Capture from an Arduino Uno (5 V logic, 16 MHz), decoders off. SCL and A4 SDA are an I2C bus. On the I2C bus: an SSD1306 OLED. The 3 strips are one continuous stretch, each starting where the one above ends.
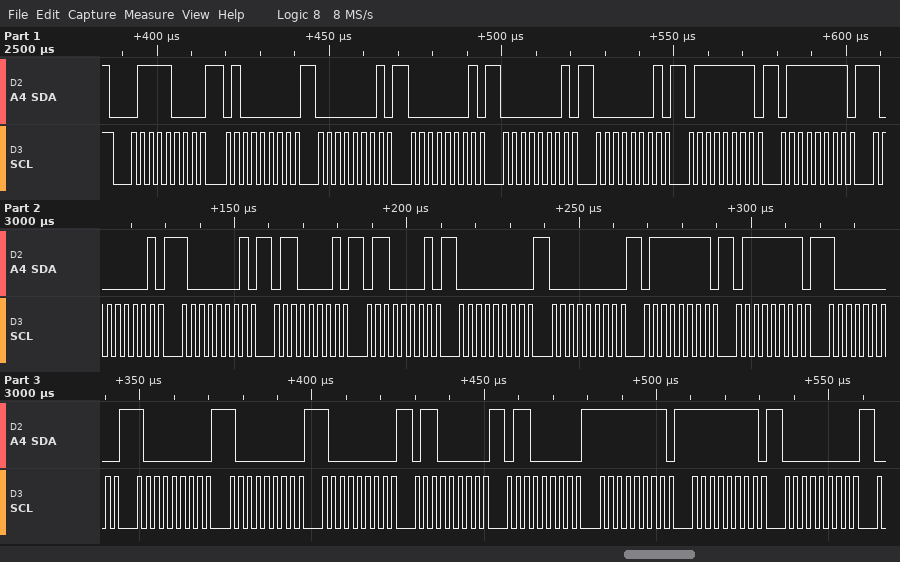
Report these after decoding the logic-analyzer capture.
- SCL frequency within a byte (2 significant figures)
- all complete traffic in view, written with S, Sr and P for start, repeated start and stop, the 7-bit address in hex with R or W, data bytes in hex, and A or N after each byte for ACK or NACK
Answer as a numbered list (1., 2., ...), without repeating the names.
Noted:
1. 400 kHz
2. S 3CW A 40 A 01 A 01 A 01 A 01 A 7F A 7F A 81 A 81 A 61 A 61 A 00 A 00 A 7F A 7F A 80 A 80 A 80 A 80 A 60 A 60 A FF A FF A 00 A
